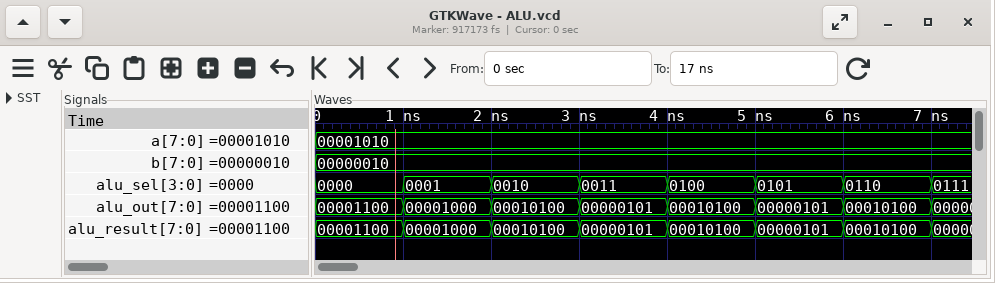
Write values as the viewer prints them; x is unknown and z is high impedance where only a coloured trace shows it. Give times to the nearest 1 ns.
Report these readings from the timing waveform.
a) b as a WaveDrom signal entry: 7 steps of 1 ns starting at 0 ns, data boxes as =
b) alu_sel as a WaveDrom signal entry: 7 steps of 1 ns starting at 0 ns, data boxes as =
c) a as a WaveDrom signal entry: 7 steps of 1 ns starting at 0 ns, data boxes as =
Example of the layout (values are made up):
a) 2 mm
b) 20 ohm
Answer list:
a) {name: 'b', wave: '=......', data: '00000010'}
b) {name: 'alu_sel', wave: '=======', data: '0000 0001 0010 0011 0100 0101 0110'}
c) {name: 'a', wave: '=......', data: '00001010'}
